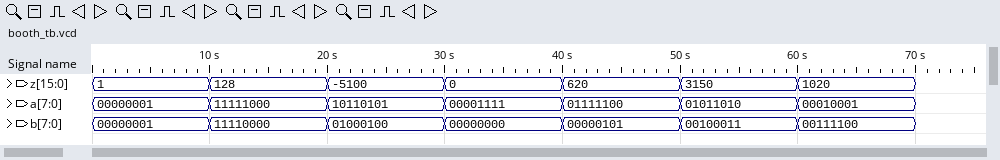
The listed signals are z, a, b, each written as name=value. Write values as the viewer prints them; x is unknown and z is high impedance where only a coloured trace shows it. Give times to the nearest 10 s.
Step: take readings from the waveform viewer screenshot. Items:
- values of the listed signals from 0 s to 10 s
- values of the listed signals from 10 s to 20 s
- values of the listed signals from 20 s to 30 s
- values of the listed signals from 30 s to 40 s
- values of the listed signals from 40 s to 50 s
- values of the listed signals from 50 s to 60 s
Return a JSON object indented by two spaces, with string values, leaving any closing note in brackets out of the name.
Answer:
{
  "values of the listed signals from 0 s to 10 s": "z=1, a=00000001, b=00000001",
  "values of the listed signals from 10 s to 20 s": "z=128, a=11111000, b=11110000",
  "values of the listed signals from 20 s to 30 s": "z=-5100, a=10110101, b=01000100",
  "values of the listed signals from 30 s to 40 s": "z=0, a=00001111, b=00000000",
  "values of the listed signals from 40 s to 50 s": "z=620, a=01111100, b=00000101",
  "values of the listed signals from 50 s to 60 s": "z=3150, a=01011010, b=00100011"
}
